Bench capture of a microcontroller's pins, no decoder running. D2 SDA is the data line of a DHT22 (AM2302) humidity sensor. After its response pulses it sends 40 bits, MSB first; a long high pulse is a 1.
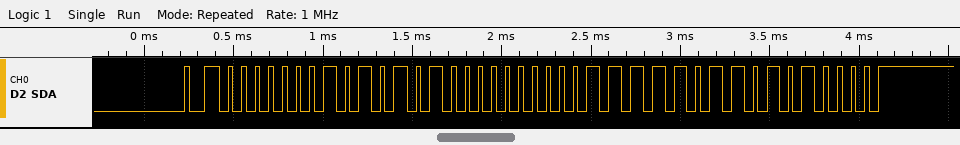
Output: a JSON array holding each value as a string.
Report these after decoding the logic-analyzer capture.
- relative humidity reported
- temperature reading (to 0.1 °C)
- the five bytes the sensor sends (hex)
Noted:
["34.0 %", "25.1 °C", "01 54 00 FB 50"]
